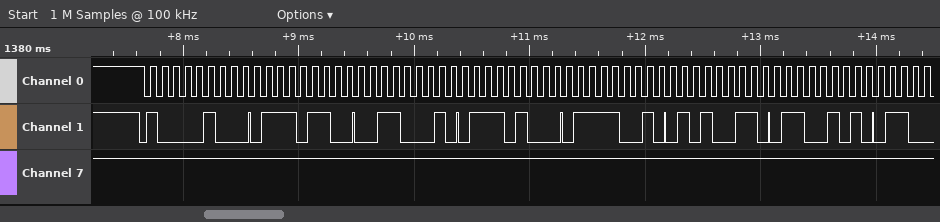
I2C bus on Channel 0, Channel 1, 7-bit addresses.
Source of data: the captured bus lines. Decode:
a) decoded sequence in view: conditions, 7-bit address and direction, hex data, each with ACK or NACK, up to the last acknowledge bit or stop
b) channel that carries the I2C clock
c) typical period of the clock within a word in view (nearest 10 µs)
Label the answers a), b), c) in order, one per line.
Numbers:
a) start, address 42 write ACK, 76 ACK, 31 ACK, 74 ACK, 79 ACK, 53 ACK, 65 ACK
b) Channel 0
c) 100 µs
